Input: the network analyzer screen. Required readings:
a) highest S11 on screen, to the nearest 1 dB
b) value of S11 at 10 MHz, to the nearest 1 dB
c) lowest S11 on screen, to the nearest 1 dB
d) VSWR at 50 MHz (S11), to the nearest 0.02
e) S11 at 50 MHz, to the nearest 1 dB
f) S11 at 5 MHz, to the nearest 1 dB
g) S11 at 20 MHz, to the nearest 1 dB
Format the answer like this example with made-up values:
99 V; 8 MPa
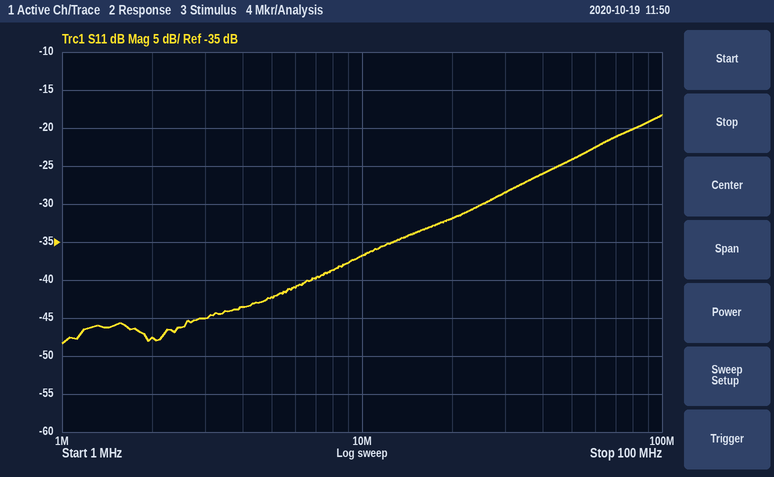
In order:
-18 dB; -37 dB; -48 dB; 1.14; -24 dB; -42 dB; -32 dB
